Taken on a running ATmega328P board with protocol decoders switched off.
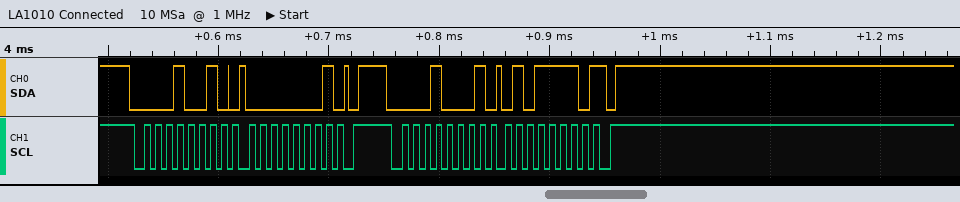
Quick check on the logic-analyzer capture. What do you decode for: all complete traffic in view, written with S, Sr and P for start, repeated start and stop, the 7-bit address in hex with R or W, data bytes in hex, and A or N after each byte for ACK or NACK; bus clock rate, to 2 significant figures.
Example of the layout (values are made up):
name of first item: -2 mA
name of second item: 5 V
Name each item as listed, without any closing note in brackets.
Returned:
all complete traffic in view, written with S, Sr and P for start, repeated start and stop, the 7-bit address in hex with R or W, data bytes in hex, and A or N after each byte for ACK or NACK: S 09W A 01 A P S 08R A 5E N P
bus clock rate, to 2 significant figures: 100 kHz
